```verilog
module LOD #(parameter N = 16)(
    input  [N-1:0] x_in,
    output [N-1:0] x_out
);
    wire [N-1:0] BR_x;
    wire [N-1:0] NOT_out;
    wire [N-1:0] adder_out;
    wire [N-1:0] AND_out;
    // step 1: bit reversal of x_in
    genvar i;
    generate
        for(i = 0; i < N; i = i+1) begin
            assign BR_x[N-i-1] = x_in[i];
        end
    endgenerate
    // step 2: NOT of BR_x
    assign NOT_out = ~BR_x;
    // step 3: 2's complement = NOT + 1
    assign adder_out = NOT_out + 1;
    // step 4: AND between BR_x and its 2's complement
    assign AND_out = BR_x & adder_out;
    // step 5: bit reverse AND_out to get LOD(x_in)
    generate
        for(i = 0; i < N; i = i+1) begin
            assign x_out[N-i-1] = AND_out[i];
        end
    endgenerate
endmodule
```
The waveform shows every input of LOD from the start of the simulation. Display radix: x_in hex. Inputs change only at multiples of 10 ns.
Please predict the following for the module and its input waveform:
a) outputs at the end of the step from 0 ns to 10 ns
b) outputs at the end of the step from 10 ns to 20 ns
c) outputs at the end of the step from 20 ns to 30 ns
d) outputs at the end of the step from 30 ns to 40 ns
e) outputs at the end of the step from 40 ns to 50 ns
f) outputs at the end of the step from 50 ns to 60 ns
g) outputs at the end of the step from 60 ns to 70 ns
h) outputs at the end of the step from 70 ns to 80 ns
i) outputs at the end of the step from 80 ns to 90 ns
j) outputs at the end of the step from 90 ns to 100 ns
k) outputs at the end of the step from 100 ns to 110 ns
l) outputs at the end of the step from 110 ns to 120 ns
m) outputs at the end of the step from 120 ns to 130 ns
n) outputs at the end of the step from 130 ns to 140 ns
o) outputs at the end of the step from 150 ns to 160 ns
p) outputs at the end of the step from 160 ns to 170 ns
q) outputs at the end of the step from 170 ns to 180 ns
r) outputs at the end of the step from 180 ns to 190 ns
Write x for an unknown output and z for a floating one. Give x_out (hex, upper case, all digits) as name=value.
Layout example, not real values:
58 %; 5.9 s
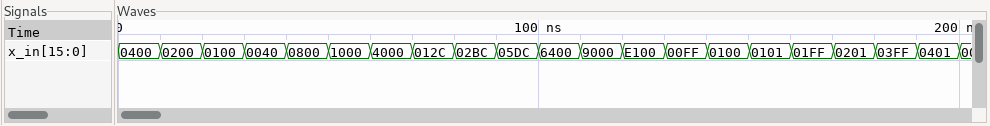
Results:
x_out=0400; x_out=0200; x_out=0100; x_out=0040; x_out=0800; x_out=1000; x_out=4000; x_out=0100; x_out=0200; x_out=0400; x_out=4000; x_out=8000; x_out=8000; x_out=0080; x_out=0100; x_out=0100; x_out=0200; x_out=0200
